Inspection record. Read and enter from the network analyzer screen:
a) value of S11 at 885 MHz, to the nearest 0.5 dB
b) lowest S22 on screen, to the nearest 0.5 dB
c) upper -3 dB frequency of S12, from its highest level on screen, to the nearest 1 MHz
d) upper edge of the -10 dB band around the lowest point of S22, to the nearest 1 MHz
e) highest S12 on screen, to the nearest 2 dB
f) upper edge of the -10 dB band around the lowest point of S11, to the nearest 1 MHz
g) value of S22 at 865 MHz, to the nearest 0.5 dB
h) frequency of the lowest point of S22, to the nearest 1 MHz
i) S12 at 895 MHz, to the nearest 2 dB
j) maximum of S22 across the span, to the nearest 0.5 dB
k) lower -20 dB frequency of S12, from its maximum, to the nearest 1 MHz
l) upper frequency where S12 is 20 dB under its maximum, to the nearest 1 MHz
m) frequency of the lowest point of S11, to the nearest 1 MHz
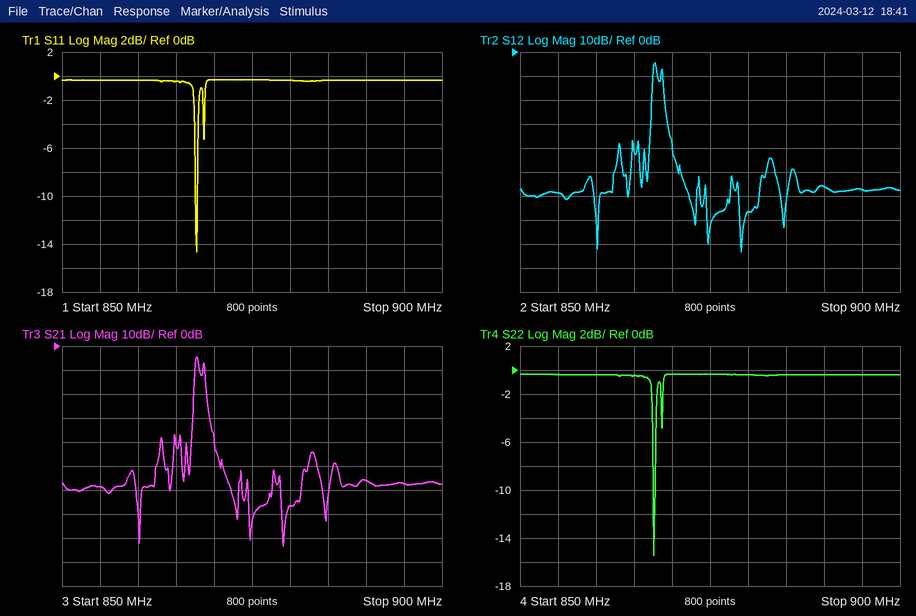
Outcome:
-0.5 dB
-15.5 dB
868 MHz
868 MHz
-4 dB
868 MHz
-0.5 dB
868 MHz
-58 dB
-0.5 dB
867 MHz
869 MHz
868 MHz
